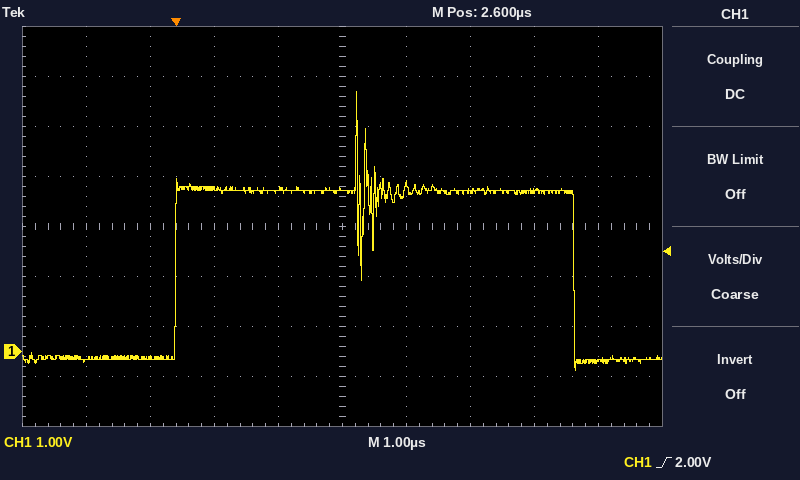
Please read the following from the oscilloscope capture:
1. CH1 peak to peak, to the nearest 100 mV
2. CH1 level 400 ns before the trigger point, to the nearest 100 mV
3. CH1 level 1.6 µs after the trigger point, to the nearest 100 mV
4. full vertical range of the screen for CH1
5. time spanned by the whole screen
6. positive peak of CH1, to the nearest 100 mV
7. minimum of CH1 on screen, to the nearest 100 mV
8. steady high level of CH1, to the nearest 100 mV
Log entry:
5.6 V
-100 mV
3.2 V
8 V
10 µs
5.2 V
-400 mV
3.2 V
